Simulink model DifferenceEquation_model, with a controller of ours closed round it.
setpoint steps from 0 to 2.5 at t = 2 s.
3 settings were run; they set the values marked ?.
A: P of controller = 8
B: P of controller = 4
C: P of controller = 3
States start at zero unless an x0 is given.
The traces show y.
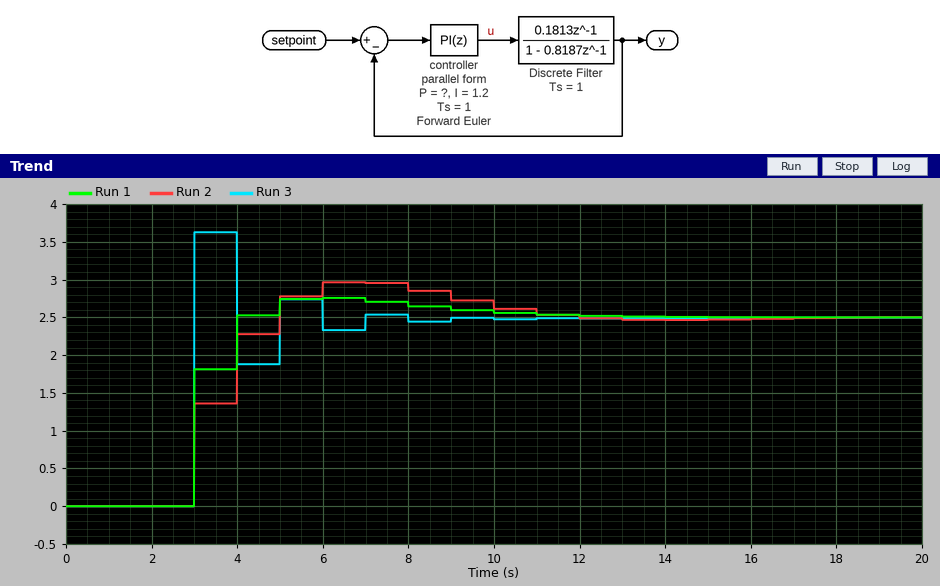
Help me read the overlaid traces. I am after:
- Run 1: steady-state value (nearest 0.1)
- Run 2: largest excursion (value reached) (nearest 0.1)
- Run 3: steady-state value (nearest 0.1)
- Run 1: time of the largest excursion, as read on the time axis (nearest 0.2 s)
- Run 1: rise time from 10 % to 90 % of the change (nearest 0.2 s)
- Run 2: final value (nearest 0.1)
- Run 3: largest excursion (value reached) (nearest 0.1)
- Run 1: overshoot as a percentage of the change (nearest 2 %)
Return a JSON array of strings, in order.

["2.5", "3.0", "2.5", "6.0 s", "1.0 s", "2.5", "3.6", "10 %"]
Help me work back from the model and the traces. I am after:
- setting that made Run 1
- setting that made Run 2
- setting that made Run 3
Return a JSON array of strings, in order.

["B", "C", "A"]
